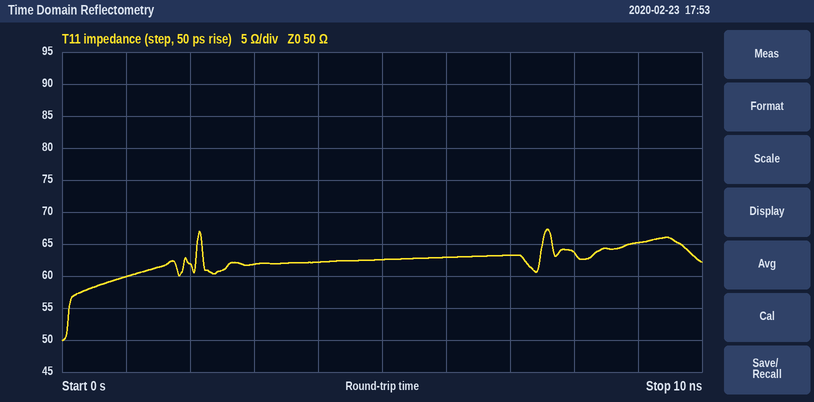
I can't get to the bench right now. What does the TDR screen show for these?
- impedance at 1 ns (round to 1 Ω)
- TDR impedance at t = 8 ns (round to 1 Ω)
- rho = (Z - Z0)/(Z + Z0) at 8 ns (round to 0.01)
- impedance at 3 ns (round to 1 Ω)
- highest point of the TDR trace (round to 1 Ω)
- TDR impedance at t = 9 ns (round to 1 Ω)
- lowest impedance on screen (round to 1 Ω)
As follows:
60 Ω
64 Ω
+0.12
62 Ω
67 Ω
65 Ω
50 Ω
